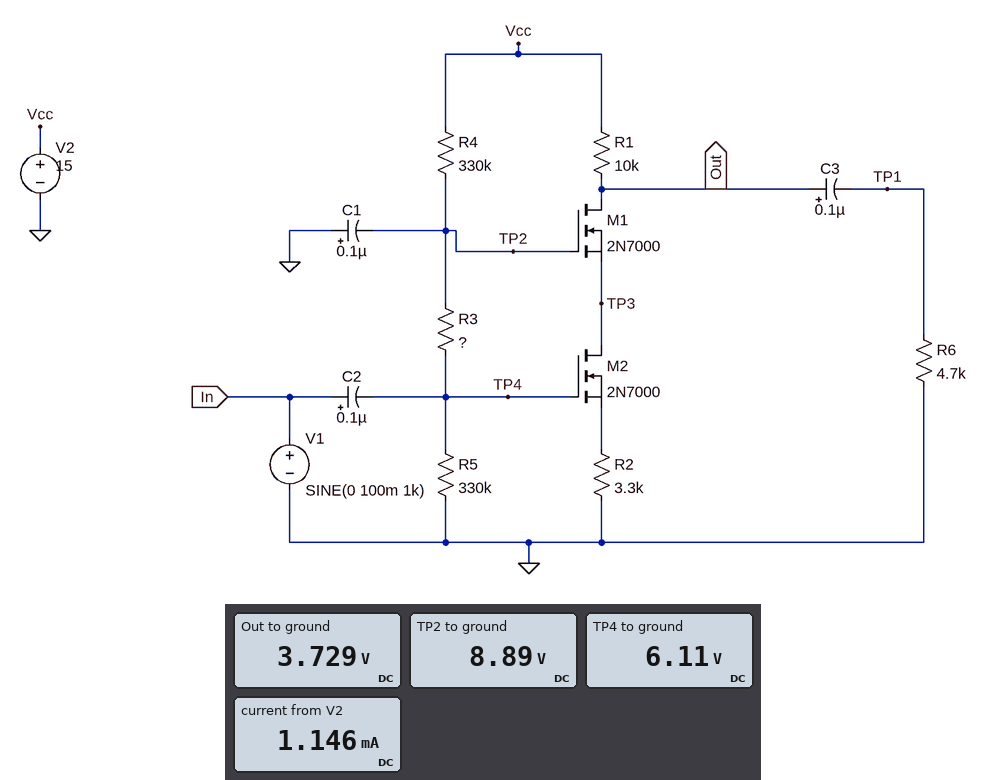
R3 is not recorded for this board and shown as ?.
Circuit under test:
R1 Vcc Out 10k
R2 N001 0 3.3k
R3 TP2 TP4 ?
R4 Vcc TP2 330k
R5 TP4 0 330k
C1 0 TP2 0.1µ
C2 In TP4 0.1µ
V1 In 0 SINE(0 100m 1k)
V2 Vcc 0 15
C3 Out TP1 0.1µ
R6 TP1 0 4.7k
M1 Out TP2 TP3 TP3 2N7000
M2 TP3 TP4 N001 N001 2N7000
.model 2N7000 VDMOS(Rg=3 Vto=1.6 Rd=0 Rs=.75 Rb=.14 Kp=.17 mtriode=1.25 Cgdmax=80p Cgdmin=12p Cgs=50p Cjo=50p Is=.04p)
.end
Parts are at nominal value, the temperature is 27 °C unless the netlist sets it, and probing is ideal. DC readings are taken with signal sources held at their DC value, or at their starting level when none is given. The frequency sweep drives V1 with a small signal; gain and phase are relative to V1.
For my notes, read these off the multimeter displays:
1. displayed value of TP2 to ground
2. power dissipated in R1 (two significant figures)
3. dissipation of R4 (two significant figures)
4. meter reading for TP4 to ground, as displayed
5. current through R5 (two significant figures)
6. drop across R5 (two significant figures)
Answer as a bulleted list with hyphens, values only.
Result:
- 8.89 V
- 13 mW
- 110 µW
- 6.11 V
- 19 µA
- 6.1 V
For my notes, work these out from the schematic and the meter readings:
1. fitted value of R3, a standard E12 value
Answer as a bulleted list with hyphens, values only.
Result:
- 150 kΩ
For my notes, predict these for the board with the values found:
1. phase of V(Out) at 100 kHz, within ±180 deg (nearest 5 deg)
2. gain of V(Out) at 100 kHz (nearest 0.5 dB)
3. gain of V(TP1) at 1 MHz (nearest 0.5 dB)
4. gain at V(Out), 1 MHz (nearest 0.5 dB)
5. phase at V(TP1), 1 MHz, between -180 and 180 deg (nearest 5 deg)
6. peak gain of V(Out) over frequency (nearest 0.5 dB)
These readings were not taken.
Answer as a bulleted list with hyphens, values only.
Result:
- 75 deg
- -18.0 dB
- -6.5 dB
- -6.5 dB
- 20 deg
- -6.0 dB
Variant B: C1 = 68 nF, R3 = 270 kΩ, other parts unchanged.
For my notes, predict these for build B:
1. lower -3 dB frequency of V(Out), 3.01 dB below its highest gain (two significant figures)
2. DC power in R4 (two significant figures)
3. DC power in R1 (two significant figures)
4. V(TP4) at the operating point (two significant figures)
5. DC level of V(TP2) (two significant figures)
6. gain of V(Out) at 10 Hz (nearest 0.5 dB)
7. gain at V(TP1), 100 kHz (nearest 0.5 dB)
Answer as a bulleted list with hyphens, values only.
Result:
- 7.6 Hz
- 86 µW
- 12 mW
- 5.3 V
- 9.7 V
- 6.5 dB
- -1.0 dB
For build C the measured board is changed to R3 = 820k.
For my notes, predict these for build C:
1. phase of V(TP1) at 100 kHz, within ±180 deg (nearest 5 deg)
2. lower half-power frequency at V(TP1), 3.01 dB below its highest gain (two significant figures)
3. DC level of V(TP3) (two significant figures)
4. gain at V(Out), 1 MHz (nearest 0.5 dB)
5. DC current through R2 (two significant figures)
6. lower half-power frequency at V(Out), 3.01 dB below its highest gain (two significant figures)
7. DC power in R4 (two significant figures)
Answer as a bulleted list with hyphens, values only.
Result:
- 160 deg
- 110 Hz
- 9.8 V
- -9.5 dB
- 520 µA
- 6.0 Hz
- 34 µW
